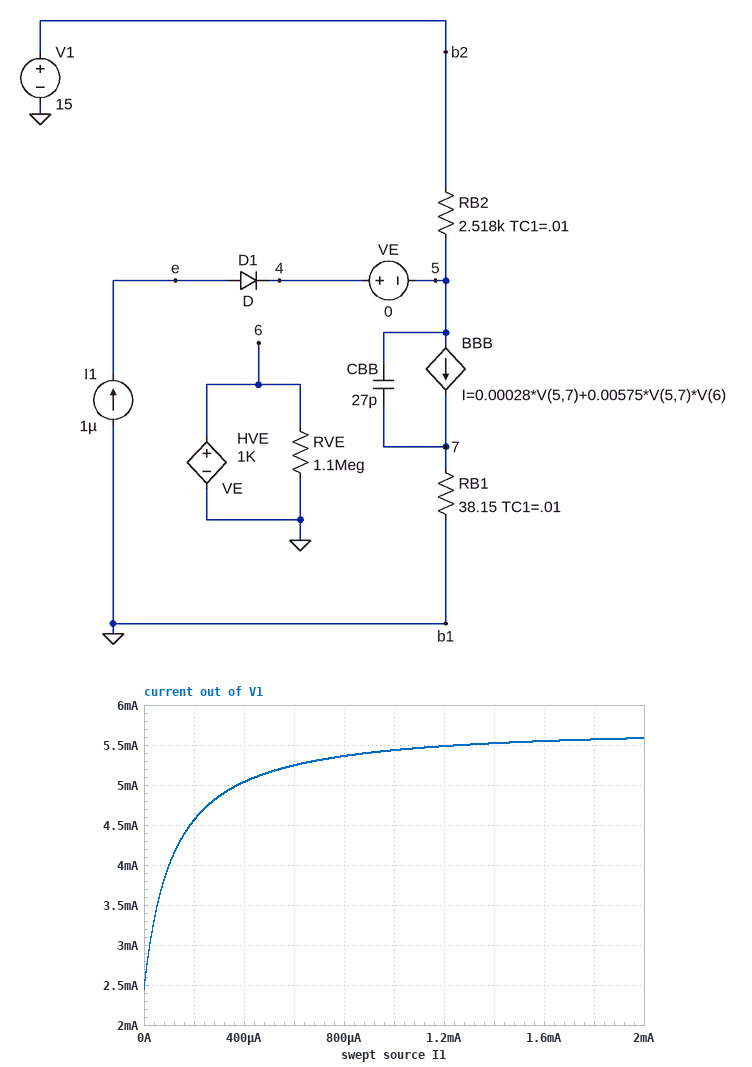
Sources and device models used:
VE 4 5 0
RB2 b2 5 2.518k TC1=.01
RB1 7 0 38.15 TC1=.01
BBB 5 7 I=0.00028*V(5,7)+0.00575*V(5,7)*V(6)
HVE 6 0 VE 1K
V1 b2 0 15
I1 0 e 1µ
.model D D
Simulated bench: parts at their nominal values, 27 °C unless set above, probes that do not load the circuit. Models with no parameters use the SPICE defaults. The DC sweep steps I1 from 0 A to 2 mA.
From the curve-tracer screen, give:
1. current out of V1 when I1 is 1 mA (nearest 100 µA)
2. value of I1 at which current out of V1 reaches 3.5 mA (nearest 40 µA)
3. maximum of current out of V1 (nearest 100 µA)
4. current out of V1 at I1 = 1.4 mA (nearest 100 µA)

5.4 mA
40 µA
5.6 mA
5.5 mA
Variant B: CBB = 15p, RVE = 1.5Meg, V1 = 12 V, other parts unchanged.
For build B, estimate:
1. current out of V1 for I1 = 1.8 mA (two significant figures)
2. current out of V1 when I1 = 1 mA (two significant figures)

4.4 mA
4.3 mA
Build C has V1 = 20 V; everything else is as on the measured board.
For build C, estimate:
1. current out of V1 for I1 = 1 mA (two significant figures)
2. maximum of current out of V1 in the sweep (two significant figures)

7.3 mA
7.5 mA
